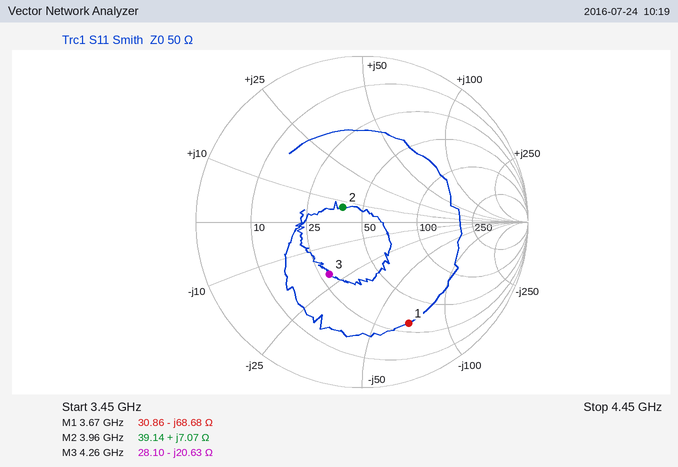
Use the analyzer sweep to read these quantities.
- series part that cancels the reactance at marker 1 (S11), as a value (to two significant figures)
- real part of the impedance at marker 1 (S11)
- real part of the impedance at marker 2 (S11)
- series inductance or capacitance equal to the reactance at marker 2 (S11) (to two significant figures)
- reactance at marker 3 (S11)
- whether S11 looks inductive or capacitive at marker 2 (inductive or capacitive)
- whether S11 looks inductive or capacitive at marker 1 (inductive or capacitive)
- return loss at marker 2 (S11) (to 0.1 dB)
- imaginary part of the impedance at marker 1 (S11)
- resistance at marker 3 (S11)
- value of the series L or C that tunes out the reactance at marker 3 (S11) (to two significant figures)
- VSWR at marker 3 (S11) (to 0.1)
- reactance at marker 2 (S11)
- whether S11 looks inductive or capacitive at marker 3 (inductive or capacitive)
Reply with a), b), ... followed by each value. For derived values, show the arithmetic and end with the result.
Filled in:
a) L = 68.68 Ω/(2π × 3.67 GHz) ≈ 3.0 nH
b) 30.86 Ω
c) 39.14 Ω
d) L = 7.07 Ω/(2π × 3.96 GHz) ≈ 284 pH, so 280 pH to two significant figures
e) -20.63 Ω
f) inductive
g) capacitive
h) 16.8 dB
i) -68.68 Ω
j) 28.10 Ω
k) L = 20.63 Ω/(2π × 4.26 GHz) ≈ 771 pH, so 770 pH to two significant figures
l) 2.2
m) +7.07 Ω
n) capacitive
